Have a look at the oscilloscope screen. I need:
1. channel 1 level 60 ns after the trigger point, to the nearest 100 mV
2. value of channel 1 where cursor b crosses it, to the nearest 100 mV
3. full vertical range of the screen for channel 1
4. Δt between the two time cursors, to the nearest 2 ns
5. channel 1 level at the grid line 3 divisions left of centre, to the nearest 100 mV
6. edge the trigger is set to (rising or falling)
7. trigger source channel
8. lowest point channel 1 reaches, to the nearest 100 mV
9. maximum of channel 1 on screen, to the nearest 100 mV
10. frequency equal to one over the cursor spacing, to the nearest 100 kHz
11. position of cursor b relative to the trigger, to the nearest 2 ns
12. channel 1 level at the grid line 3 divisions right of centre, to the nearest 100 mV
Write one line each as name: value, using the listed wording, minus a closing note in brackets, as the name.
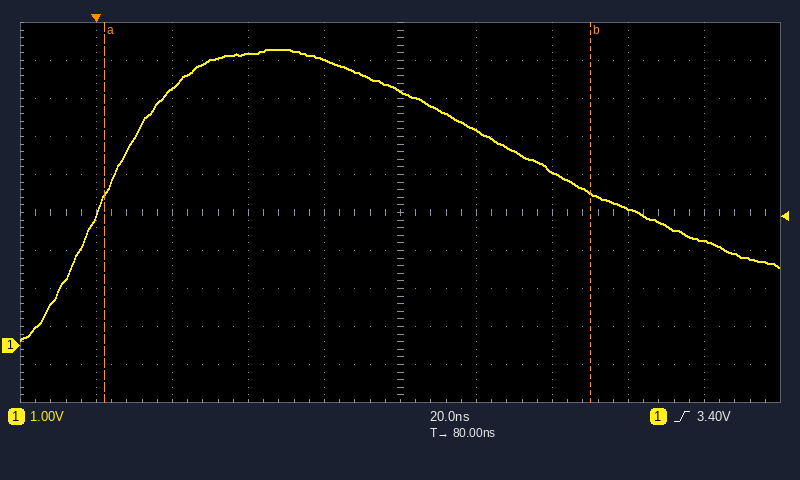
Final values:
channel 1 level 60 ns after the trigger point, to the nearest 100 mV: 7.5 V
value of channel 1 where cursor b crosses it, to the nearest 100 mV: 4.0 V
full vertical range of the screen for channel 1: 10 V
Δt between the two time cursors, to the nearest 2 ns: 128 ns
channel 1 level at the grid line 3 divisions left of centre, to the nearest 100 mV: 6.8 V
edge the trigger is set to: rising
trigger source channel: channel 1
lowest point channel 1 reaches, to the nearest 100 mV: 100 mV
maximum of channel 1 on screen, to the nearest 100 mV: 7.8 V
frequency equal to one over the cursor spacing, to the nearest 100 kHz: 7.8 MHz
position of cursor b relative to the trigger, to the nearest 2 ns: +130 ns
channel 1 level at the grid line 3 divisions right of centre, to the nearest 100 mV: 3.6 V
